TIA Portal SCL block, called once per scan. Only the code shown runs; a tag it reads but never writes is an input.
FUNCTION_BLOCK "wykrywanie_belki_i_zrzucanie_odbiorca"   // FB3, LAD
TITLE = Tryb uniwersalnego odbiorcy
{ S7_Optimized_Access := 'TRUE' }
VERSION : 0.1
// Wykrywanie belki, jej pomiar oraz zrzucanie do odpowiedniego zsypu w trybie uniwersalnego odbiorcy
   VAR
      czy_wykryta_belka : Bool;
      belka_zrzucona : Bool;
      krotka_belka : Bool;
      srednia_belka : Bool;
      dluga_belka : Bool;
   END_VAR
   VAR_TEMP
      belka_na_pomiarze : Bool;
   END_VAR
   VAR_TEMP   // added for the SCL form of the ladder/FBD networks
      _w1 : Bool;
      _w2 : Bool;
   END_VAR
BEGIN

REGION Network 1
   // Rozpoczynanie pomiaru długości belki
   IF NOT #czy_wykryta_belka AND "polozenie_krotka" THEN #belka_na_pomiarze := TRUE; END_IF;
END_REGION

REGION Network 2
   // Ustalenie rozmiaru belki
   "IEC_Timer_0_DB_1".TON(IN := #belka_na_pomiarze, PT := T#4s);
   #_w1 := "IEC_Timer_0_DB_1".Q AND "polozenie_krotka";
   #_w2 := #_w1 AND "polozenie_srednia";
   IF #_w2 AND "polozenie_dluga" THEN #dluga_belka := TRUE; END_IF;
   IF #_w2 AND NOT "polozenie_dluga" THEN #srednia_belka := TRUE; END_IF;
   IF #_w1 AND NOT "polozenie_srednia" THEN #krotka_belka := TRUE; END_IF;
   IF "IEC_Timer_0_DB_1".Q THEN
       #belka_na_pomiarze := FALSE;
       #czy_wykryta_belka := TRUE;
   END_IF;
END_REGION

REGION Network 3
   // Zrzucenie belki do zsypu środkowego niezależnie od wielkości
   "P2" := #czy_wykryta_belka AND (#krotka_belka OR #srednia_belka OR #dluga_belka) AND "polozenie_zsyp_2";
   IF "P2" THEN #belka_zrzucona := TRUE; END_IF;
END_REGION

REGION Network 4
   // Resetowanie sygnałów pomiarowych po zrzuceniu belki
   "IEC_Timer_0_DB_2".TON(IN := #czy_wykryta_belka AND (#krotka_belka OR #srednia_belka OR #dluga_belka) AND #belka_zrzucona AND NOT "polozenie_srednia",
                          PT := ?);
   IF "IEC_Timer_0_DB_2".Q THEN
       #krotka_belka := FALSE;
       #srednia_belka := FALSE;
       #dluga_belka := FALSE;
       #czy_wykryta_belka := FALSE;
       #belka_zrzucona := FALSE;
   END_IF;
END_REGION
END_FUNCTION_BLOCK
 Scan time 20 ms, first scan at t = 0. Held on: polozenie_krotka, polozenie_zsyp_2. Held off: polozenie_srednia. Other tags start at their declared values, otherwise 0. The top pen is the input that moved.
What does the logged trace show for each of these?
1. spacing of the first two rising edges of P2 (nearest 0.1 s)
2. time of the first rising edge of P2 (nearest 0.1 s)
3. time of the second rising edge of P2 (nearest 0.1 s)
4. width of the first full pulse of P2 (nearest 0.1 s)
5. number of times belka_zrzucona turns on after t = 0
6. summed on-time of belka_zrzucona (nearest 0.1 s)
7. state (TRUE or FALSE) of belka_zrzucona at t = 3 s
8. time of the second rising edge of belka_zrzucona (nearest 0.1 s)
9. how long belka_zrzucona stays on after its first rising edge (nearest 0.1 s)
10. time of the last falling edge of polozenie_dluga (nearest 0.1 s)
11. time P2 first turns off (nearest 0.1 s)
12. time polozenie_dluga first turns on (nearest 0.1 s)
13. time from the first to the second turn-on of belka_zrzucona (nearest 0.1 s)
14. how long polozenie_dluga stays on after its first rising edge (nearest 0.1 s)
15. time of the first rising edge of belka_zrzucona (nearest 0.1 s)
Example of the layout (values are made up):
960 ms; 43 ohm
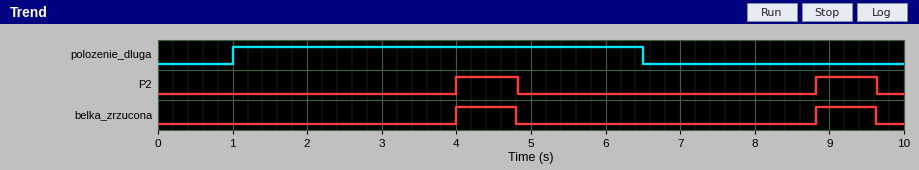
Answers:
4.8 s; 4.0 s; 8.8 s; 0.8 s; 2; 1.6 s; FALSE; 8.8 s; 0.8 s; 6.5 s; 4.8 s; 1.0 s; 4.8 s; 5.5 s; 4.0 s
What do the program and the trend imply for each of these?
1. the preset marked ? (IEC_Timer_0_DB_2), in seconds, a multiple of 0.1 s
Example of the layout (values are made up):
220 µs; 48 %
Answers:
0.8 s
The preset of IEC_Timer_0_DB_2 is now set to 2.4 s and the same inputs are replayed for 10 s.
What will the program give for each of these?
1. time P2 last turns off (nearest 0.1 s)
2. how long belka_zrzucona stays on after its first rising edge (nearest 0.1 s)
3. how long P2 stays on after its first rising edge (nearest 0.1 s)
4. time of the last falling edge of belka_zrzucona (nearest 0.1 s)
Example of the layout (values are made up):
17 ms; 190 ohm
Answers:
6.4 s; 2.4 s; 2.4 s; 6.4 s
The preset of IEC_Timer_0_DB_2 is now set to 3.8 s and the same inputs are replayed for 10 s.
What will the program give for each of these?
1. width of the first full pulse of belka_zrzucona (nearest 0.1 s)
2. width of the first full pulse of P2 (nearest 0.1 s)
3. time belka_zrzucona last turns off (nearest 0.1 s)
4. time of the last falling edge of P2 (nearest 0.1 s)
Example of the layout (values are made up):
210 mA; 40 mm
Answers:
3.8 s; 3.8 s; 7.8 s; 7.8 s
